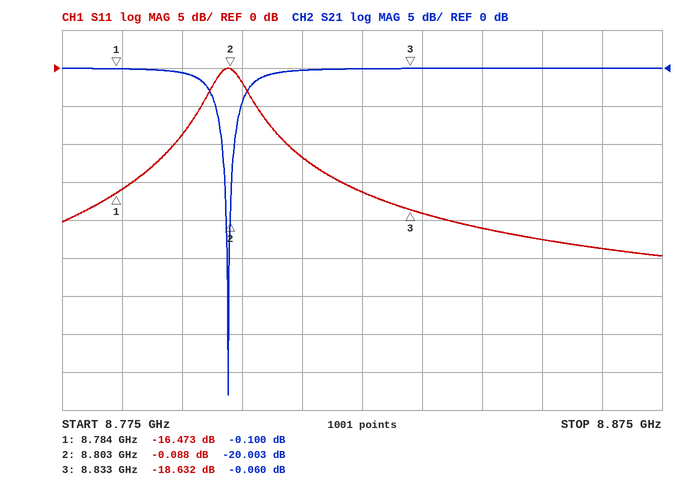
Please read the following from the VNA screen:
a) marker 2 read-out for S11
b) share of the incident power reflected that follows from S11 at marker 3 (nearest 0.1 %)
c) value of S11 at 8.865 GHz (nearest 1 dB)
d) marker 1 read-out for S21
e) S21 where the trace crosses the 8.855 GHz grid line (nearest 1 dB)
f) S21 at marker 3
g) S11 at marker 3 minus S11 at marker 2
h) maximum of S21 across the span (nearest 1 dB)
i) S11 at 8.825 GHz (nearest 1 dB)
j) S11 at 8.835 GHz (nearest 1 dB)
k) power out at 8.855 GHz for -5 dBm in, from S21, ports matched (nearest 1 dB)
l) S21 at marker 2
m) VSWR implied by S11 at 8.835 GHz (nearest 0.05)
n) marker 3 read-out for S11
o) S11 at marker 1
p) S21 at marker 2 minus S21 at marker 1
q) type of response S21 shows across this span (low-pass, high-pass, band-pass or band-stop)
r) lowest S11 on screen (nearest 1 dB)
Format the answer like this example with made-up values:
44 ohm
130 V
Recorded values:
-0.088 dB
1.4 %
-24 dB
-0.100 dB
0 dB
-0.060 dB
-18.544 dB
0 dB
-16 dB
-19 dB
-5 dBm
-20.003 dB
1.25
-18.632 dB
-16.473 dB
-19.903 dB
band-stop
-25 dB
